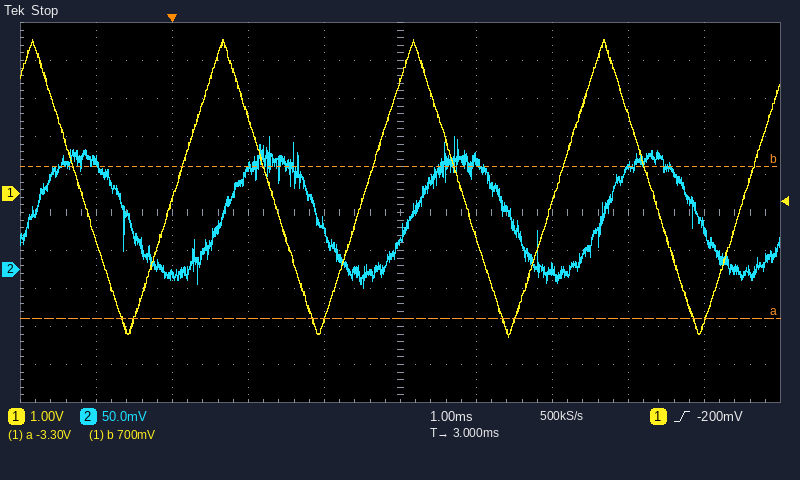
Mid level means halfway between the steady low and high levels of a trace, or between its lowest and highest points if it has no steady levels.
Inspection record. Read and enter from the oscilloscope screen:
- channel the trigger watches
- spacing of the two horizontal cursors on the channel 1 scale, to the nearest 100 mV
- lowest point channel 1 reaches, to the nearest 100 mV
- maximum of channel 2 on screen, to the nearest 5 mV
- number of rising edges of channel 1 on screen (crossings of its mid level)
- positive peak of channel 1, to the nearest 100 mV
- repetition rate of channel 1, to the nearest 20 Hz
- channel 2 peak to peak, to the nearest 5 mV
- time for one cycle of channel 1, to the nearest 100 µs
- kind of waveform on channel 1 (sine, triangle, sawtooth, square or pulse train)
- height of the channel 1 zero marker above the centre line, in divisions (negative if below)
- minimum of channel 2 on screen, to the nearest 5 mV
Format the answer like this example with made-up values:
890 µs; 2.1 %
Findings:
channel 1; 4.0 V; -3.8 V; 175 mV; 4; 4.1 V; 400 Hz; 200 mV; 2.5 ms; triangle; +0.5 div; -25 mV
